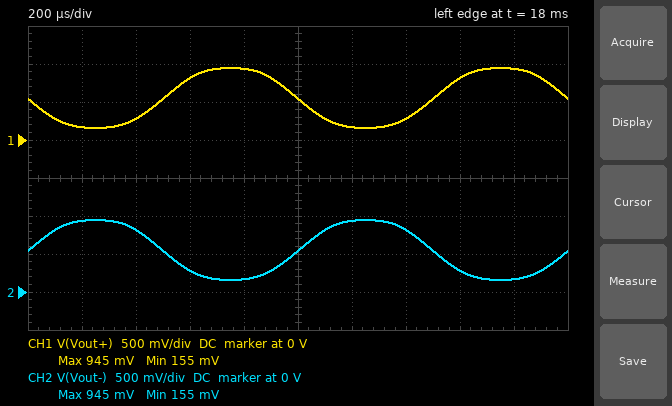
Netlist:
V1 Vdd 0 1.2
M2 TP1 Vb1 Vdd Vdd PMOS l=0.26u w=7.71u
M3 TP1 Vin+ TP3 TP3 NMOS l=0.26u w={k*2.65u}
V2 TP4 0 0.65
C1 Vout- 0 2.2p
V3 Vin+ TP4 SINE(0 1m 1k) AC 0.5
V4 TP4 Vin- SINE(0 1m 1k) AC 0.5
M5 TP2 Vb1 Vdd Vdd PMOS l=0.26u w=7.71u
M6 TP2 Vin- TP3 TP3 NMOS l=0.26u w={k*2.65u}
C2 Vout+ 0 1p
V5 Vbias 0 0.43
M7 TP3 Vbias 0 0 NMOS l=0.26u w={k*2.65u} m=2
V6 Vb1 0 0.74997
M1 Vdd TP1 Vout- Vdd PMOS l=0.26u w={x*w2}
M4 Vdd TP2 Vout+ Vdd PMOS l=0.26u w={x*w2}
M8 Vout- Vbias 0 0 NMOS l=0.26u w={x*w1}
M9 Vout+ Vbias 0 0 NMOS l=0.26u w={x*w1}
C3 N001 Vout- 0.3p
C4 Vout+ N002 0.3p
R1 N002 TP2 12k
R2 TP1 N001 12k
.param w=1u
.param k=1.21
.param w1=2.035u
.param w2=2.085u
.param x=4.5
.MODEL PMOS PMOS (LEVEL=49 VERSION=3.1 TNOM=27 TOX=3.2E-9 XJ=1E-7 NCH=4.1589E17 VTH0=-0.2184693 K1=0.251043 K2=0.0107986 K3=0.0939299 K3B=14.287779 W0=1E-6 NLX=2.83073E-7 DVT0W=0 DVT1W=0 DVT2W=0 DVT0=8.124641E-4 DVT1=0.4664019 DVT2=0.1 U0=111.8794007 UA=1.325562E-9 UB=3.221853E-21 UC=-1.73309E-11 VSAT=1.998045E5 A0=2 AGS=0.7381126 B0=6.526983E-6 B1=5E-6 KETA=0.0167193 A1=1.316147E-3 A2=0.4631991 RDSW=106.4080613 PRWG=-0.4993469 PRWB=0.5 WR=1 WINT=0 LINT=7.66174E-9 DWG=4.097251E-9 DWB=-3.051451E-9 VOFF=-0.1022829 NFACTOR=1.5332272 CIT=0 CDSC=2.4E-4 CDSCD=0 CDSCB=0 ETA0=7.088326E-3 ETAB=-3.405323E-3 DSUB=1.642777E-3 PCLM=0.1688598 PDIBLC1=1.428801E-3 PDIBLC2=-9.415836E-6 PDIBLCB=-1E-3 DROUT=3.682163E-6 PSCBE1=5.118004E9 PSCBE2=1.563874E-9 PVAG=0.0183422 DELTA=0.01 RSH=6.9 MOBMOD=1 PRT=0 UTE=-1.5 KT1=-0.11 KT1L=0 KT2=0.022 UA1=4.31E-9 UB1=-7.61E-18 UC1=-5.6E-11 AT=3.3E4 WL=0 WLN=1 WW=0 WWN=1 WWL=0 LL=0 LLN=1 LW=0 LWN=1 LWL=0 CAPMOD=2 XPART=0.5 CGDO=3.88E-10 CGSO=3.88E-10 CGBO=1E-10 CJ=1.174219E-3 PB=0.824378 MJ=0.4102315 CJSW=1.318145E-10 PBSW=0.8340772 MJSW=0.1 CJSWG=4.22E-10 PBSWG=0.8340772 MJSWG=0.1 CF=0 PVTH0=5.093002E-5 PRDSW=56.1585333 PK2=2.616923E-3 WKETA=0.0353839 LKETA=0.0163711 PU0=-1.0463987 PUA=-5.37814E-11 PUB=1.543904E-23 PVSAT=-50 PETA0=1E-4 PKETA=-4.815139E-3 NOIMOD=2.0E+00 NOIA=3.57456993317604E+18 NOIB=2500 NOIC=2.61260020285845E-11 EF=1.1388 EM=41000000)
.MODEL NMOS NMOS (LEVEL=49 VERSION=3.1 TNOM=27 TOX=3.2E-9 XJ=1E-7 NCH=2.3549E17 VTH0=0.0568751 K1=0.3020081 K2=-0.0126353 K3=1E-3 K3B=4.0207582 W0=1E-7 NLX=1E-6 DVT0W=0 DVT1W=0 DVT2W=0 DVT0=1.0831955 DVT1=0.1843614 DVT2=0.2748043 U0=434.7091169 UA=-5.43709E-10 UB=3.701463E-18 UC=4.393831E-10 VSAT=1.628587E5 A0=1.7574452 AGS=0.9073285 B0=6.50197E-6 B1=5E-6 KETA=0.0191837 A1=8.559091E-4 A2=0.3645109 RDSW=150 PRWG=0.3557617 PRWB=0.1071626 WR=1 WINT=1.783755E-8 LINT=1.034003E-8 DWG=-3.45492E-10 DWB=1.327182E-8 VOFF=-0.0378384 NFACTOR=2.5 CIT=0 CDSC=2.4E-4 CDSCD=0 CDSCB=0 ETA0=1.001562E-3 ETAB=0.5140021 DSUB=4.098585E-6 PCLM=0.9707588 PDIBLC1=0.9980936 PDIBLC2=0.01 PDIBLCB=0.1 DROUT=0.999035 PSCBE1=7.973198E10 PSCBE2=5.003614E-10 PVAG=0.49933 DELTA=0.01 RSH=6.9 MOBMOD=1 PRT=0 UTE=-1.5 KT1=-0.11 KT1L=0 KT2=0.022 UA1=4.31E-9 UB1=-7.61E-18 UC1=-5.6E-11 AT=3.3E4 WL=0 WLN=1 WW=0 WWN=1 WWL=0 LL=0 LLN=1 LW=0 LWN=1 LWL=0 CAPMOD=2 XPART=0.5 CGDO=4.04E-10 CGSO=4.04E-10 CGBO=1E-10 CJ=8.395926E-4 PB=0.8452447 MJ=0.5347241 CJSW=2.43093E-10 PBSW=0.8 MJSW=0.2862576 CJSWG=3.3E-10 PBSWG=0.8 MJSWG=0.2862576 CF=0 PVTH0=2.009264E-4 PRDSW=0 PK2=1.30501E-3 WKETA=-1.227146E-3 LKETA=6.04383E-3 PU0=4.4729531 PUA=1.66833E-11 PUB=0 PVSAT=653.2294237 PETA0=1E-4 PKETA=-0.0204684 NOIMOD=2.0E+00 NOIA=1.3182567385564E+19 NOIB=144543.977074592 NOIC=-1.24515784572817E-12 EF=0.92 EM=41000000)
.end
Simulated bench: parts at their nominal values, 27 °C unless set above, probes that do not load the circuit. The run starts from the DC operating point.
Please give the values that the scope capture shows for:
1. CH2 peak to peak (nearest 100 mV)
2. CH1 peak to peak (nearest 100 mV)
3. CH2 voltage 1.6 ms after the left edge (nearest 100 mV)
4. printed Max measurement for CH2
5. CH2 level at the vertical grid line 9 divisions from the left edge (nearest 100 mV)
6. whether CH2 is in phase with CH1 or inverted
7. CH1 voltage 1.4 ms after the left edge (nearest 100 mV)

800 mV
800 mV
300 mV
945 mV
200 mV
inverted
300 mV
